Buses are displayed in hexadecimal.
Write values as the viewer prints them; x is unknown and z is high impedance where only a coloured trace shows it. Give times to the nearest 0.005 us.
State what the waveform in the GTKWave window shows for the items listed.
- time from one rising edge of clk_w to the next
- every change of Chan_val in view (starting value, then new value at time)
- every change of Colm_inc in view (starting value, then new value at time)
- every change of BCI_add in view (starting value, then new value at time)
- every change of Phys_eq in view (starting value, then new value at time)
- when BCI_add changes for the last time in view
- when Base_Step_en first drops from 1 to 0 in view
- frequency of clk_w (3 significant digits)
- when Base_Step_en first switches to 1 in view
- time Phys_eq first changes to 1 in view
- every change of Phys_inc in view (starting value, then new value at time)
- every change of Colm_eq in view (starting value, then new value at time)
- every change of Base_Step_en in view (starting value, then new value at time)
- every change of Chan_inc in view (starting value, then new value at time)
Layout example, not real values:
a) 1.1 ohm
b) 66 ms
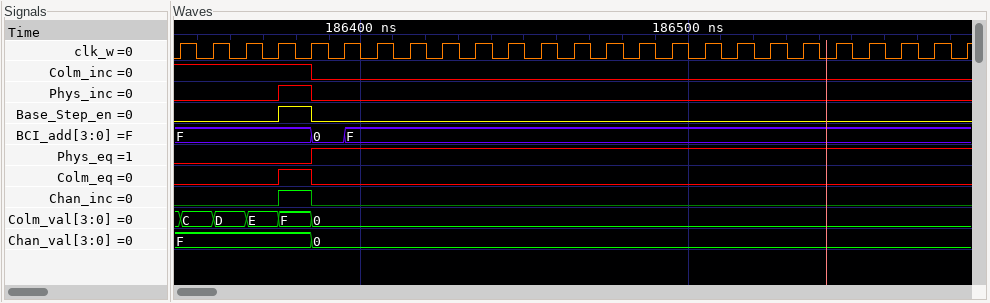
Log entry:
a) 0.01 us
b) F, 0 at 186.385 us
c) 1, 0 at 186.385 us
d) F, 0 at 186.385 us, F at 186.395 us
e) 0, 1 at 186.385 us
f) 186.395 us
g) 186.385 us
h) 100 MHz
i) 186.375 us
j) 186.385 us
k) 0, 1 at 186.375 us, 0 at 186.385 us
l) 0, 1 at 186.375 us, 0 at 186.385 us
m) 0, 1 at 186.375 us, 0 at 186.385 us
n) 0, 1 at 186.375 us, 0 at 186.385 us
